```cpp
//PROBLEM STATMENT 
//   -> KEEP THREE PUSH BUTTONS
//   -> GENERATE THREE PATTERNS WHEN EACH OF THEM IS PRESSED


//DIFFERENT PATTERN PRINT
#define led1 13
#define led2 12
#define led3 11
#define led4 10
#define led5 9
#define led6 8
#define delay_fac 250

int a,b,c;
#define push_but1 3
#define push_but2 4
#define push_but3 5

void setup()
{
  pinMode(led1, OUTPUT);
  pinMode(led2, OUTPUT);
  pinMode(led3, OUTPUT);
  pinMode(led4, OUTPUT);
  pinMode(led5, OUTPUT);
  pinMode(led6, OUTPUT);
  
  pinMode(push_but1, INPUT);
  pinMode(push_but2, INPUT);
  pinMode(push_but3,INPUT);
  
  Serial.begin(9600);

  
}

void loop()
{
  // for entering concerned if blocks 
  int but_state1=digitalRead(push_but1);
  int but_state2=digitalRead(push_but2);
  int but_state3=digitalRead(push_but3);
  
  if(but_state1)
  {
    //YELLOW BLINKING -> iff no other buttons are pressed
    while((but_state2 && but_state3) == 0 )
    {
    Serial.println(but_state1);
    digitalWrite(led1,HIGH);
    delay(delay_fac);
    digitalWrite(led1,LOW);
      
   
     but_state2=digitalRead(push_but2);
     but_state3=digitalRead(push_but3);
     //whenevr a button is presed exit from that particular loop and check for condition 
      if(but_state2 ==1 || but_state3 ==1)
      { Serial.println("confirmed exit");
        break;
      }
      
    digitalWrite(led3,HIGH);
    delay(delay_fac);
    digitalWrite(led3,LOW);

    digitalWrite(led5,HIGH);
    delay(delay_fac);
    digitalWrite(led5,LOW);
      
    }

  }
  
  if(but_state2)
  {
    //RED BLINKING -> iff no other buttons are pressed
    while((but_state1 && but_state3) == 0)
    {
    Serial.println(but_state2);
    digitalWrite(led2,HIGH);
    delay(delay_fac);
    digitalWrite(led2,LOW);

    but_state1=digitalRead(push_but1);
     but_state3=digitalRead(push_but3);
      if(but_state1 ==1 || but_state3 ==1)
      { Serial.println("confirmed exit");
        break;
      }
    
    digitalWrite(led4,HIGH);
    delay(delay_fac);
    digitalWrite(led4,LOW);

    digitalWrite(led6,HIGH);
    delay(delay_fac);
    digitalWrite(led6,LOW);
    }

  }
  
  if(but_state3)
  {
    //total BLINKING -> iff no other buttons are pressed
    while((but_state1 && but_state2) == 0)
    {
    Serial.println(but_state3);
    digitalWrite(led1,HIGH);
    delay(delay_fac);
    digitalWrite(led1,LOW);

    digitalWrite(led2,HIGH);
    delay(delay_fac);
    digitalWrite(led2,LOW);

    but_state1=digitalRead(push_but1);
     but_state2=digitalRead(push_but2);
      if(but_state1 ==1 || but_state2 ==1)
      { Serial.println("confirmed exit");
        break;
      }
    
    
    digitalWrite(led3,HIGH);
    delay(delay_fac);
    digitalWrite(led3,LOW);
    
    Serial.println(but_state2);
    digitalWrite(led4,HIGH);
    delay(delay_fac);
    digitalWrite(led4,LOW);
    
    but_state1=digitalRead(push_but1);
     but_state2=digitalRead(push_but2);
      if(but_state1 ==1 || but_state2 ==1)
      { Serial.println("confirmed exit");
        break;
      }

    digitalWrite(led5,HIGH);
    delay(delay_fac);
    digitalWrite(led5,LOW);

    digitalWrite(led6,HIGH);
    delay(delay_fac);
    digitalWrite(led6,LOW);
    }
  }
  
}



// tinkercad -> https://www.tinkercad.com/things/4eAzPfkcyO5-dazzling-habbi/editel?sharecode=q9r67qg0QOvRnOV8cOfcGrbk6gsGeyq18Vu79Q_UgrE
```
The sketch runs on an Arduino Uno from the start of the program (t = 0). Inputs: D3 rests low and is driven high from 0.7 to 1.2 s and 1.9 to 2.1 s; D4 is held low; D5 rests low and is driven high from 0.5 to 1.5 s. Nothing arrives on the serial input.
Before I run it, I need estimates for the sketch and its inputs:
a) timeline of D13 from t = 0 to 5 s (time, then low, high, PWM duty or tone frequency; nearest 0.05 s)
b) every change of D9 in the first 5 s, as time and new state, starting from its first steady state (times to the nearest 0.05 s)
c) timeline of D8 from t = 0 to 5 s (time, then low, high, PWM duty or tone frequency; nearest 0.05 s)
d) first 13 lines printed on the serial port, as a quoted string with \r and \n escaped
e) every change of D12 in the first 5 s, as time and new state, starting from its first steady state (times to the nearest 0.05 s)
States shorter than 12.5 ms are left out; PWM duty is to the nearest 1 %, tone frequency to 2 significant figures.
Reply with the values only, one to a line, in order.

0 s low; 0.5 s high; 0.75 s low; 1 s high; 1.5 s low; 2.75 s high; 3 s low; 4.25 s high; 4.5 s low
0 s low; 2.25 s high; 2.5 s low; 3.75 s high; 4 s low
0 s low; 2.5 s high; 2.75 s low; 4 s high; 4.25 s low
"1\r\nconfirmed exit\r\n1\r\nconfirmed exit\r\n1\r\n0\r\n1\r\n0\r\n1\r\n0\r\n1\r\n0\r\n1\r\n"
0 s low; 0.75 s high; 1 s low; 1.5 s high; 1.75 s low; 3 s high; 3.25 s low; 4.5 s high; 4.75 s low
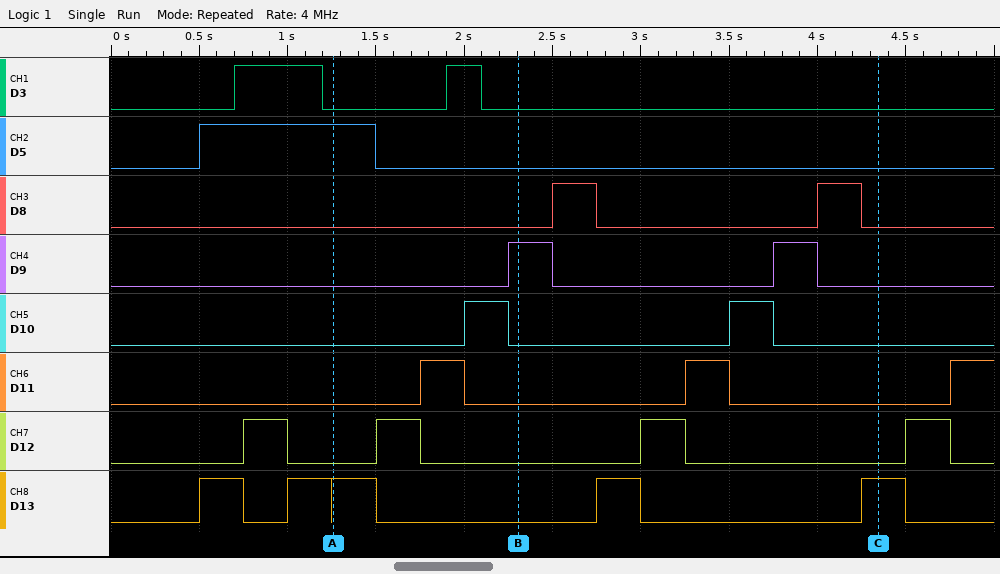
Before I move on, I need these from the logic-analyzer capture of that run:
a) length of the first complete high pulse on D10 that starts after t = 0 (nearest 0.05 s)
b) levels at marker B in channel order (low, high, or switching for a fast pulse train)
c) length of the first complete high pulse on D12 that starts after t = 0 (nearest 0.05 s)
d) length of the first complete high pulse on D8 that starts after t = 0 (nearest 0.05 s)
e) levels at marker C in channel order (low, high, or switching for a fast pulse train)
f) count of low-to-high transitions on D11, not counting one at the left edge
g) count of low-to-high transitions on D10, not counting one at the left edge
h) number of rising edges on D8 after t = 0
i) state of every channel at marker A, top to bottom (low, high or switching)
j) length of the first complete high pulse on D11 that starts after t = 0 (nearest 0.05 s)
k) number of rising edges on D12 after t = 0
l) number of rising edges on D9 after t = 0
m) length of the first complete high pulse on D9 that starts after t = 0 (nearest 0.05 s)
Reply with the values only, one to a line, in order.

0.25 s
D3 low, D5 low, D8 low, D9 high, D10 low, D11 low, D12 low, D13 low
0.25 s
0.25 s
D3 low, D5 low, D8 low, D9 low, D10 low, D11 low, D12 low, D13 high
3
2
2
D3 low, D5 high, D8 low, D9 low, D10 low, D11 low, D12 low, D13 high
0.25 s
4
2
0.25 s
